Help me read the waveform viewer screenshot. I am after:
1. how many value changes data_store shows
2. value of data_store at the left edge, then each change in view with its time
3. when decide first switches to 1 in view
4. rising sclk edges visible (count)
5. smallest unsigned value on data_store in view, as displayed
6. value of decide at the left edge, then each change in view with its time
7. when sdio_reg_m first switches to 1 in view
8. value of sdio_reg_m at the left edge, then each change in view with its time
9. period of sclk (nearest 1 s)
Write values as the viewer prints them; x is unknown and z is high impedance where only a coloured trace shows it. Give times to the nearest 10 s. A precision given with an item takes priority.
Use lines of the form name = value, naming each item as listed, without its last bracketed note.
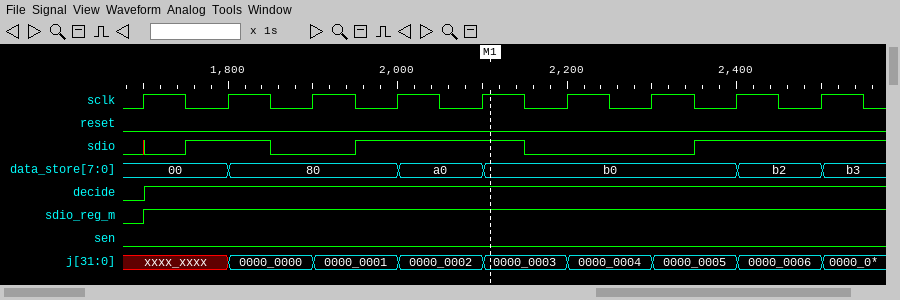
how many value changes data_store shows = 5
value of data_store at the left edge, then each change in view with its time = 00, 80 at 1800 s, a0 at 2000 s, b0 at 2100 s, b2 at 2400 s, b3 at 2500 s
when decide first switches to 1 in view = 1700 s
rising sclk edges visible = 9
smallest unsigned value on data_store in view, as displayed = 00
value of decide at the left edge, then each change in view with its time = 0, 1 at 1700 s
when sdio_reg_m first switches to 1 in view = 1700 s
value of sdio_reg_m at the left edge, then each change in view with its time = 0, 1 at 1700 s
period of sclk = 100 s
